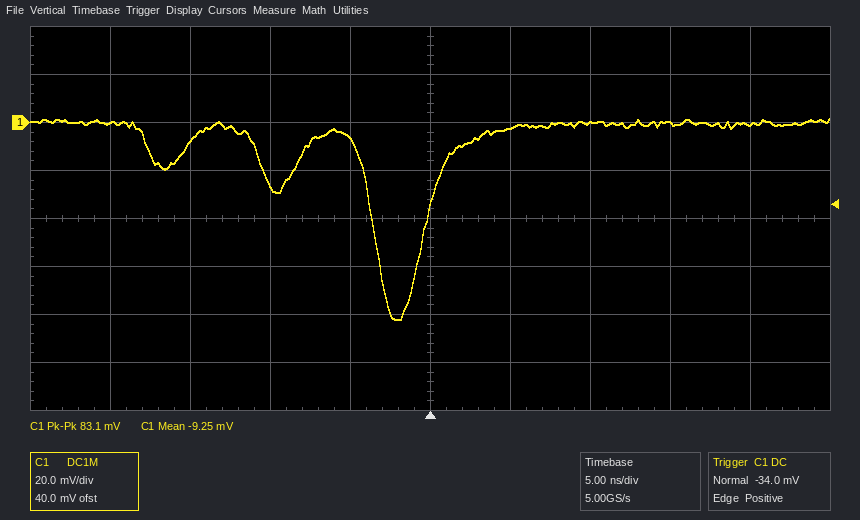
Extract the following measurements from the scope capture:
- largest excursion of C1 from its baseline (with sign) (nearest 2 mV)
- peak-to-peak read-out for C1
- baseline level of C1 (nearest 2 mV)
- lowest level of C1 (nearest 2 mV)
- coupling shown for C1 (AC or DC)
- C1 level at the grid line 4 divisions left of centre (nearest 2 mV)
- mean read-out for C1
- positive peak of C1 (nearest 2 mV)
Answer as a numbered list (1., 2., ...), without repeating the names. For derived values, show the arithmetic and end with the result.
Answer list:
1. -82 mV − (0 mV) = -82 mV
2. 83.1 mV
3. 0 mV
4. -82 mV
5. DC
6. 0 mV
7. -9.25 mV
8. 2 mV
